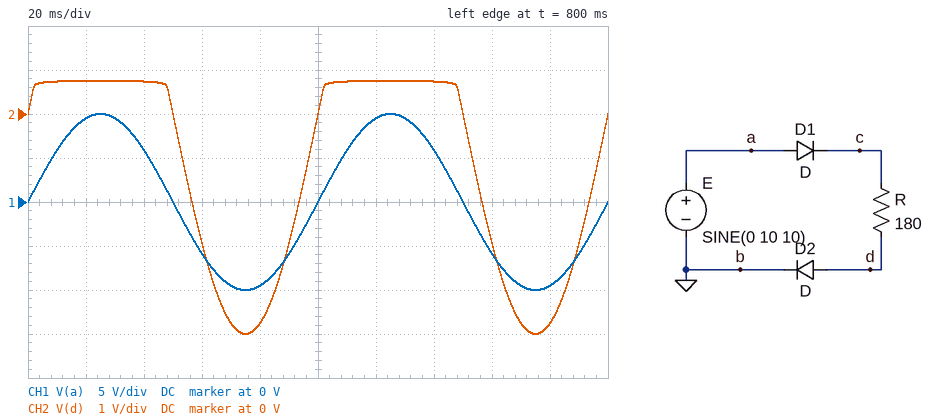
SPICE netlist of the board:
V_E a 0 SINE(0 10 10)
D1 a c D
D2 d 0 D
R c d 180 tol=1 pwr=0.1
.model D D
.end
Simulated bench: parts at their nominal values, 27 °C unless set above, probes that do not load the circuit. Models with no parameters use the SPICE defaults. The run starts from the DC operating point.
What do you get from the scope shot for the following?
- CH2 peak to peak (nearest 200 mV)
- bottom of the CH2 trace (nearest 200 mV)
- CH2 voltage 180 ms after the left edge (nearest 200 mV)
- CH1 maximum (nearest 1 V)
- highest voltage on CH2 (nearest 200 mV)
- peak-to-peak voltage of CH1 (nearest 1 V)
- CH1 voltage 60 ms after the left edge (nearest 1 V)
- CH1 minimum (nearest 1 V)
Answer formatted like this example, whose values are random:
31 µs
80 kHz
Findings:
5.8 V
-5.0 V
-4.8 V
10 V
800 mV
20 V
-6 V
-10 V
